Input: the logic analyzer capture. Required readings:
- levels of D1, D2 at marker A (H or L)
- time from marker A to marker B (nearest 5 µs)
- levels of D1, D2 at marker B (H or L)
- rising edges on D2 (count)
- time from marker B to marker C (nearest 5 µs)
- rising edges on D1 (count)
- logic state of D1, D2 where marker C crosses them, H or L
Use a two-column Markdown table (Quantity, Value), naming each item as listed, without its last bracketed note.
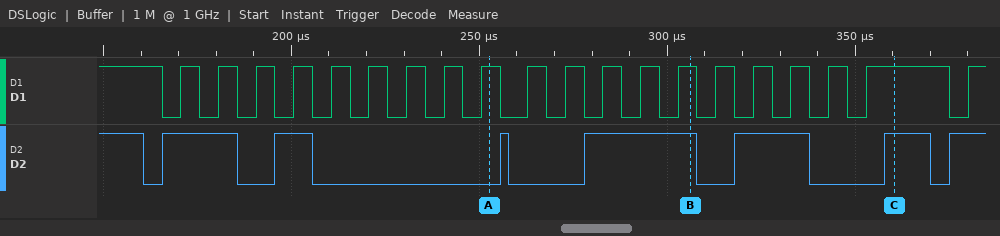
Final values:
| Quantity | Value |
|---|---|
| levels of D1, D2 at marker A | D1=H, D2=L |
| time from marker A to marker B | 55 µs |
| levels of D1, D2 at marker B | D1=H, D2=H |
| rising edges on D2 | 7 |
| time from marker B to marker C | 55 µs |
| rising edges on D1 | 20 |
| logic state of D1, D2 where marker C crosses them, H or L | D1=H, D2=H |
